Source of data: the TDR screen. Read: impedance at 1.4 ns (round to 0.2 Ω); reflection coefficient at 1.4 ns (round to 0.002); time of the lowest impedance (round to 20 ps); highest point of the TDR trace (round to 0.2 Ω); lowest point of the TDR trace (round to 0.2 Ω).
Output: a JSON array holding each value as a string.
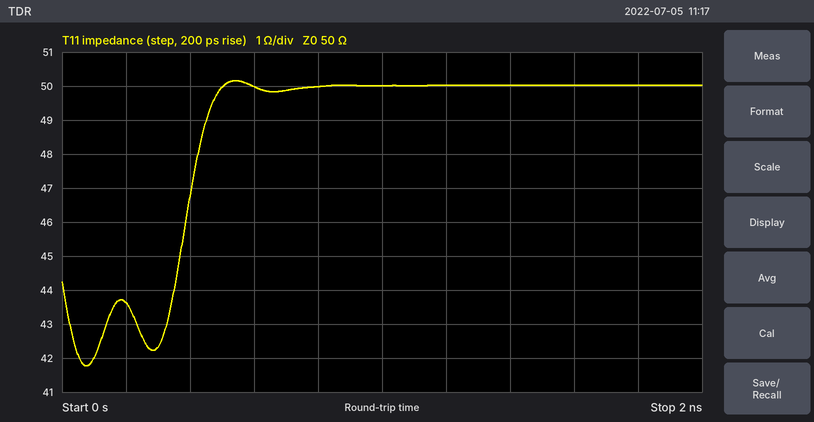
["50.0 Ω", "0.000", "80 ps", "50.2 Ω", "41.8 Ω"]
